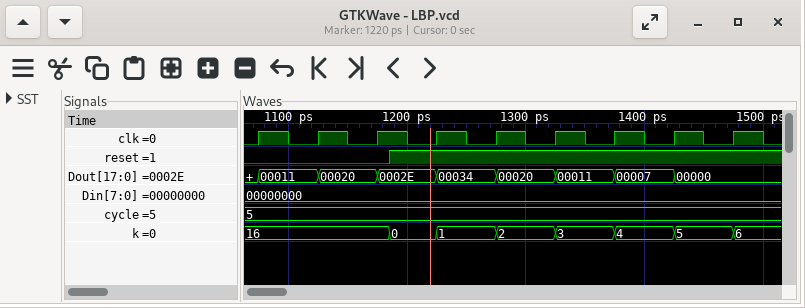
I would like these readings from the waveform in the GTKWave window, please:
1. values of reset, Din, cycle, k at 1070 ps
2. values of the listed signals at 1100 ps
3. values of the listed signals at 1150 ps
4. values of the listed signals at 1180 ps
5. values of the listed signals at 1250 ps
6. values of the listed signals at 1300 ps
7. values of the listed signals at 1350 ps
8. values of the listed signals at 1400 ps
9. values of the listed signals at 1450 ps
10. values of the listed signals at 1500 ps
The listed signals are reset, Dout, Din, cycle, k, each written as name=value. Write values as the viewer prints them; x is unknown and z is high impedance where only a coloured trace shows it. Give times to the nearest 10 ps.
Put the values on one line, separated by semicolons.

reset=0, Din=00000000, cycle=5, k=16; reset=0, Dout=00011, Din=00000000, cycle=5, k=16; reset=0, Dout=00020, Din=00000000, cycle=5, k=16; reset=0, Dout=0002E, Din=00000000, cycle=5, k=16; reset=1, Dout=00034, Din=00000000, cycle=5, k=1; reset=1, Dout=00020, Din=00000000, cycle=5, k=2; reset=1, Dout=00011, Din=00000000, cycle=5, k=3; reset=1, Dout=00007, Din=00000000, cycle=5, k=4; reset=1, Dout=00000, Din=00000000, cycle=5, k=5; reset=1, Dout=00000, Din=00000000, cycle=5, k=6
